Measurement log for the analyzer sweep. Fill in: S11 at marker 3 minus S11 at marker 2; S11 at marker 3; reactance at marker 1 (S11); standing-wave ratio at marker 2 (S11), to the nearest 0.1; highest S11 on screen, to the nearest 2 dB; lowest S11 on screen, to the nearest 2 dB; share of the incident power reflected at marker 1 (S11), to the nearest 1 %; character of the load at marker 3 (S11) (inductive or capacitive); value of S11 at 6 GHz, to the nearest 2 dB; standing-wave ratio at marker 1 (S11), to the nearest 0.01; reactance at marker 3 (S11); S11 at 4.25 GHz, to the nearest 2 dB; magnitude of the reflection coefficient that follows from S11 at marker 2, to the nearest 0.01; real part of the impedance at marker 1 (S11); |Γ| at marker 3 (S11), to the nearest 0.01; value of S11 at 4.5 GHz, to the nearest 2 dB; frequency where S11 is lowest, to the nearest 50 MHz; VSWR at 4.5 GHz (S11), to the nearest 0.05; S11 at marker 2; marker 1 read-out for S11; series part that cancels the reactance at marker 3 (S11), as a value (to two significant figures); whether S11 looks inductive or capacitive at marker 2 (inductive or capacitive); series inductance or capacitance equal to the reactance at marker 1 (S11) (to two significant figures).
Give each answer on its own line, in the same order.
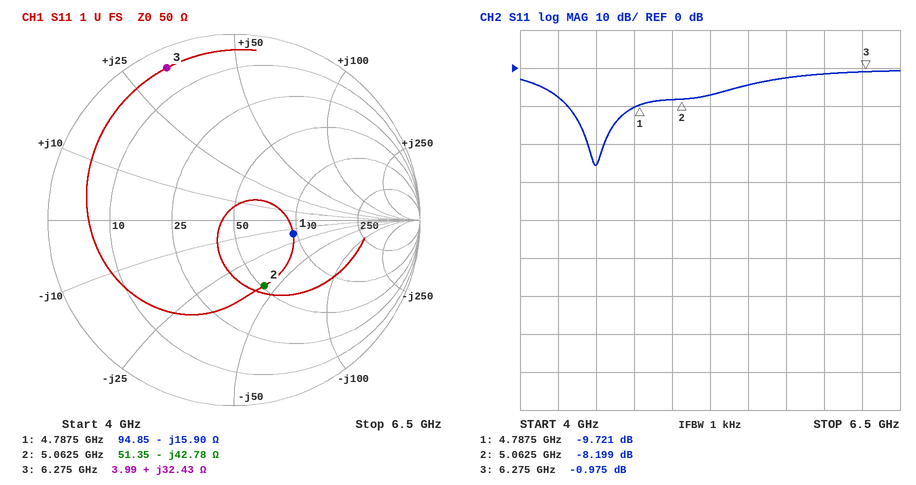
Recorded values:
7.224 dB
-0.975 dB
-15.90 Ω
2.3
0 dB
-26 dB
11 %
inductive
-2 dB
1.97
+32.43 Ω
-8 dB
0.39
94.85 Ω
0.89
-26 dB
4.50 GHz
1.10
-8.199 dB
-9.721 dB
780 fF
capacitive
2.1 pF
